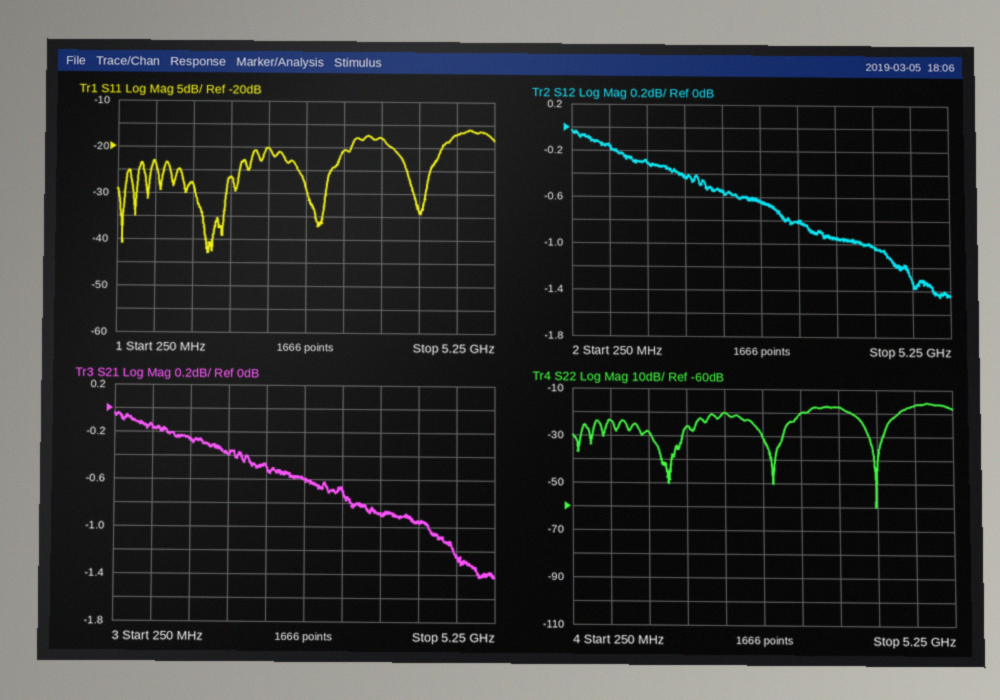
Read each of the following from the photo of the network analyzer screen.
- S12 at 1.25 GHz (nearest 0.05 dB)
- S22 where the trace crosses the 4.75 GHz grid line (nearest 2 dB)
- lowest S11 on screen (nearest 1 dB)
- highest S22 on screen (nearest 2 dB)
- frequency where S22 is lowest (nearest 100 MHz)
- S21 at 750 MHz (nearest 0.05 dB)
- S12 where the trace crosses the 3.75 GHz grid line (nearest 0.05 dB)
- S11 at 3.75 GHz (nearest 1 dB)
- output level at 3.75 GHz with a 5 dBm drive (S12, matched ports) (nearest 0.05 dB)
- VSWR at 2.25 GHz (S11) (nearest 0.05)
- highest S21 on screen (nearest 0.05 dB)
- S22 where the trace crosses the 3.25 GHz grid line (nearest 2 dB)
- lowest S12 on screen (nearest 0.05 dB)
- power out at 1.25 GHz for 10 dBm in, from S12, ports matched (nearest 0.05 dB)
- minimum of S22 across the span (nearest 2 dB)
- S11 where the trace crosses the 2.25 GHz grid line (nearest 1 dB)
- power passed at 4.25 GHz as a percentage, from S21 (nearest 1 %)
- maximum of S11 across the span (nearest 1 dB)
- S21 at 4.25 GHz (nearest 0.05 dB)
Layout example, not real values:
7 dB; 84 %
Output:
-0.30 dB; -16 dB; -43 dB; -16 dB; 4.2 GHz; -0.15 dB; -0.95 dB; -18 dB; 4.05 dBm; 1.20; -0.05 dB; -20 dB; -1.45 dB; 9.70 dBm; -60 dB; -20 dB; 80 %; -16 dB; -0.95 dB
